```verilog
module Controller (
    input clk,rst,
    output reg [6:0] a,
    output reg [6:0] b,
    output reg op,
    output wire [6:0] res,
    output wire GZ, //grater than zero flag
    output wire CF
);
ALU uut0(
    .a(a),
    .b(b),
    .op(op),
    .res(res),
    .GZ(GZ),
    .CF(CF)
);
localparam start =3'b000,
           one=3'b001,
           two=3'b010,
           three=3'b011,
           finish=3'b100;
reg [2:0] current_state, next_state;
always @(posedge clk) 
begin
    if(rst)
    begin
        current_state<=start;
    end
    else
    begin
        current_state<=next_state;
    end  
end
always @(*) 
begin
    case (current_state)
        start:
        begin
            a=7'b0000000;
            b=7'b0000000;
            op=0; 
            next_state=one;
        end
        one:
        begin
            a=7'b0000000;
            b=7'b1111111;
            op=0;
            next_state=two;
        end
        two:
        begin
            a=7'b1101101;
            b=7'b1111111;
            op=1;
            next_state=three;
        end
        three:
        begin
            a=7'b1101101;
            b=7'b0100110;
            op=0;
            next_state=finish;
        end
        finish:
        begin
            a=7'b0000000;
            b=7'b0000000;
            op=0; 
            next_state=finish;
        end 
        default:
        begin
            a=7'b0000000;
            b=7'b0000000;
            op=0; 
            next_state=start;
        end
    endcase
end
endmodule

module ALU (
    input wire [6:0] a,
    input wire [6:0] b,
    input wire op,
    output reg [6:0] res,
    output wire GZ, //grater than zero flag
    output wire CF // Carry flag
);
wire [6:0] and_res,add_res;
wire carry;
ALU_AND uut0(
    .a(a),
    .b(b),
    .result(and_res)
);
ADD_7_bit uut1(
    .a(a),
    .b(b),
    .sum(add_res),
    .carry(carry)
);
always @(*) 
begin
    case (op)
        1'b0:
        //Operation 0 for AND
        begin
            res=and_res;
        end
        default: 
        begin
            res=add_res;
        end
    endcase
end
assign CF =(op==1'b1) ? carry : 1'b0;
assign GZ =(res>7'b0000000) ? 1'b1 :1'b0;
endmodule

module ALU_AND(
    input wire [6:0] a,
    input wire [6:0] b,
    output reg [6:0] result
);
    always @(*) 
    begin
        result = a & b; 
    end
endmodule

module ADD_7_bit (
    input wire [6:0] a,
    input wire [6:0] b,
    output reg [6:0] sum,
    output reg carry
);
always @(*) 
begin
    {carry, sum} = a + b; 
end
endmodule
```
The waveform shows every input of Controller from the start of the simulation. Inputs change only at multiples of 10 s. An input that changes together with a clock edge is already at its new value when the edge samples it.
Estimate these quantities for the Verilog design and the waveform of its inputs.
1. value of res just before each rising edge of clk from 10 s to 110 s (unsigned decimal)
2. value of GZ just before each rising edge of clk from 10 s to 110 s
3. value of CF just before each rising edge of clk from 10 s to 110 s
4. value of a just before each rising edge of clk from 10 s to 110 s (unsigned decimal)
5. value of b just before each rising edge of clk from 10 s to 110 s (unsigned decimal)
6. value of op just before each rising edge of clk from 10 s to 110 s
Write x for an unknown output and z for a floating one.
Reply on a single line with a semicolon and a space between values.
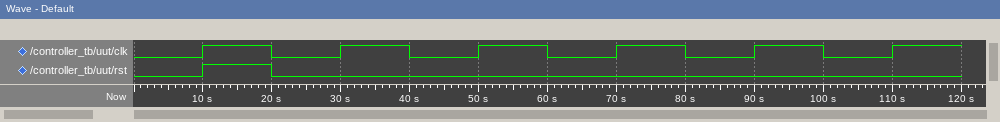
x, 0, 0, 108, 36, 0; x 0 0 1 1 0; x 0 0 1 0 0; x, 0, 0, 109, 109, 0; x, 0, 127, 127, 38, 0; x 0 0 1 0 0
